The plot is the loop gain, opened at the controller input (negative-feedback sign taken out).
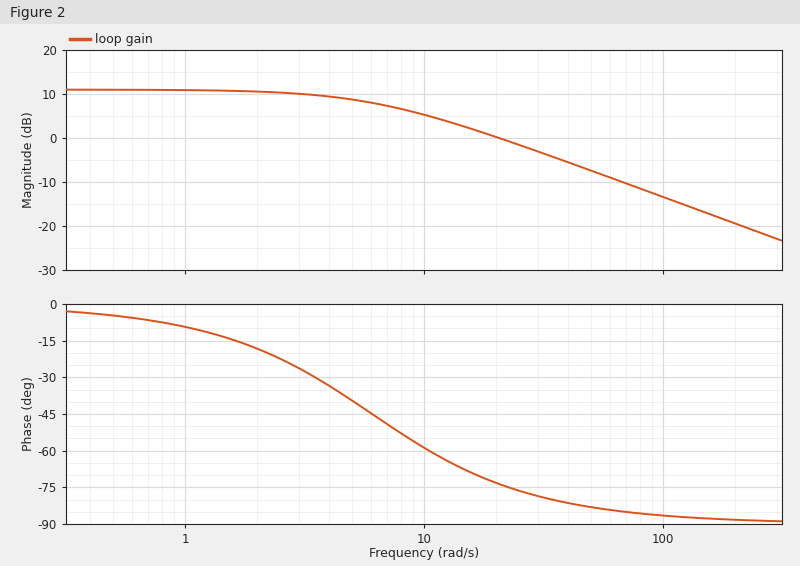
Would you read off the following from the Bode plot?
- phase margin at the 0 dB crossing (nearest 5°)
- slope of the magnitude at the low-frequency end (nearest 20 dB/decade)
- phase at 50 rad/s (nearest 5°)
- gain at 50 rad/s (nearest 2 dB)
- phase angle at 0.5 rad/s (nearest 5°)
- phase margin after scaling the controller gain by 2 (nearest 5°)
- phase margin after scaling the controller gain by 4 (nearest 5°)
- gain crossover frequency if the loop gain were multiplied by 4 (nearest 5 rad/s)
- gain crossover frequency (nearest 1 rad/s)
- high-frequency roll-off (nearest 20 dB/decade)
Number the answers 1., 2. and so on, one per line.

1. 105°
2. 0 dB/decade
3. -85°
4. -8 dB
5. -5°
6. 100°
7. 95°
8. 85 rad/s
9. 21 rad/s
10. -20 dB/decade
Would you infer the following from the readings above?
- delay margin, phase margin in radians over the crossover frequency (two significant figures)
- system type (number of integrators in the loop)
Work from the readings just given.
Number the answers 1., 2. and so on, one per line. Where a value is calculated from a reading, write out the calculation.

1. 105 × π / 180 / 21 = 0.087 s
2. 0
